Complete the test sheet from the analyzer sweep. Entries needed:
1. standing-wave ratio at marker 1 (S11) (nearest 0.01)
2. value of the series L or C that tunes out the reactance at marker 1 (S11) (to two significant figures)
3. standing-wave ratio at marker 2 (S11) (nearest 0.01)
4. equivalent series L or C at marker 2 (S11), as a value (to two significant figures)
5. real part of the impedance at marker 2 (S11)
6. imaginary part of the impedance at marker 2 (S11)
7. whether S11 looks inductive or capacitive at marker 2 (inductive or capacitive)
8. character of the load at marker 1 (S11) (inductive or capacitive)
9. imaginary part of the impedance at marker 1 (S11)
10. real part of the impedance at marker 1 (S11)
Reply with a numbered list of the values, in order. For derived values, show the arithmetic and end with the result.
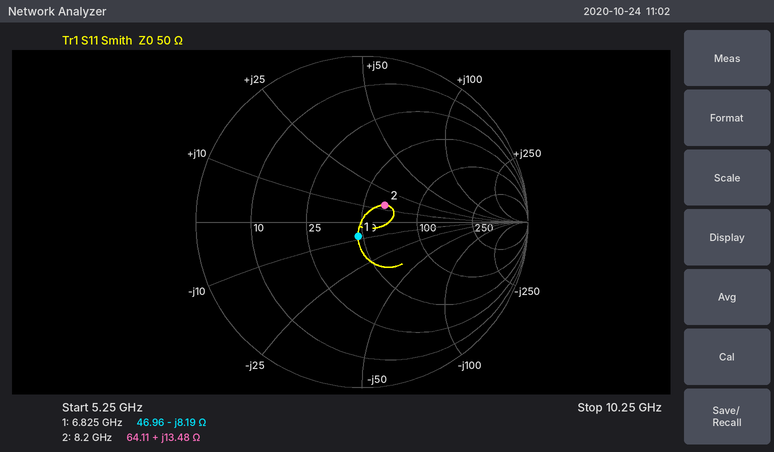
1. 1.20
2. L = 8.19 Ω/(2π × 6.825 GHz) ≈ 191 pH, so 190 pH to two significant figures
3. 1.41
4. L = 13.48 Ω/(2π × 8.2 GHz) ≈ 262 pH, so 260 pH to two significant figures
5. 64.11 Ω
6. +13.48 Ω
7. inductive
8. capacitive
9. -8.19 Ω
10. 46.96 Ω
